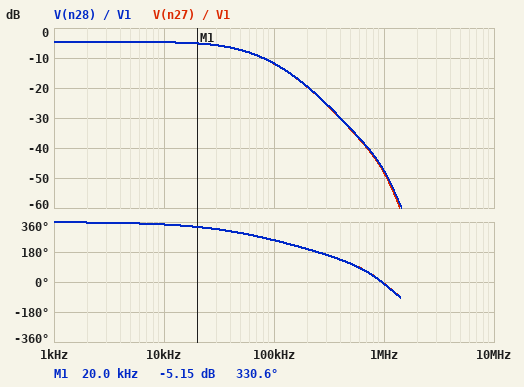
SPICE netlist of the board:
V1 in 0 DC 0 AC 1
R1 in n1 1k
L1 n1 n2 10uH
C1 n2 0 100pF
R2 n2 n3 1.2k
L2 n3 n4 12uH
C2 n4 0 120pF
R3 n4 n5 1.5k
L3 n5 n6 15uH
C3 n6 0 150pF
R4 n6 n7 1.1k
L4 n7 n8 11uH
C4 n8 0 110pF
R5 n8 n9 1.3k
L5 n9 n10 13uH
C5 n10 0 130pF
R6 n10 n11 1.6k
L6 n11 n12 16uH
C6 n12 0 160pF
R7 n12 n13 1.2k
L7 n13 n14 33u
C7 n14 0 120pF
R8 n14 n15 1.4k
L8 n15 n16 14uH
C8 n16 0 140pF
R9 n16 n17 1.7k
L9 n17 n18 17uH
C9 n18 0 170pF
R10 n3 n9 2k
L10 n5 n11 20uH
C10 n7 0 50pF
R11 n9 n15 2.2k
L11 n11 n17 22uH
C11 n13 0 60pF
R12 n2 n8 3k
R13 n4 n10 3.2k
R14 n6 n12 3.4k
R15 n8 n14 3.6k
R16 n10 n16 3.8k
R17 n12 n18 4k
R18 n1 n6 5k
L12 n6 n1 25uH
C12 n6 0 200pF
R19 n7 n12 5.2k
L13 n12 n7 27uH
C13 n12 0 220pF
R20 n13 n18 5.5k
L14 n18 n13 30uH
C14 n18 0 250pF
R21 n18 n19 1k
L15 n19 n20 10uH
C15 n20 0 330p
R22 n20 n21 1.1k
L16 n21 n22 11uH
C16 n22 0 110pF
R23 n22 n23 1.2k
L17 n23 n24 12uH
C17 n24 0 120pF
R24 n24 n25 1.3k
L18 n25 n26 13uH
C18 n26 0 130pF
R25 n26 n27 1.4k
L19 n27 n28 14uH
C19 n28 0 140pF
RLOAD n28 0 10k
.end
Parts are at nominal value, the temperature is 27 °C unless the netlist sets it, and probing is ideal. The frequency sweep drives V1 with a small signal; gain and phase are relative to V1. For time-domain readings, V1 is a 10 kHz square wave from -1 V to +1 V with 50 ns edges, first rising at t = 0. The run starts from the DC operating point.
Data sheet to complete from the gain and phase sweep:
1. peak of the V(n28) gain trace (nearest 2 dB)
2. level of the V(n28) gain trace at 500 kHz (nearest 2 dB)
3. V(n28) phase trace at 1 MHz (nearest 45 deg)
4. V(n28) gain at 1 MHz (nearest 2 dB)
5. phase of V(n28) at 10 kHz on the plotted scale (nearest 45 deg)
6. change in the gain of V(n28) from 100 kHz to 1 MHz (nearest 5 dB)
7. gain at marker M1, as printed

-4 dB
-34 dB
0 deg
-48 dB
360 deg
-35 dB
-5.15 dB
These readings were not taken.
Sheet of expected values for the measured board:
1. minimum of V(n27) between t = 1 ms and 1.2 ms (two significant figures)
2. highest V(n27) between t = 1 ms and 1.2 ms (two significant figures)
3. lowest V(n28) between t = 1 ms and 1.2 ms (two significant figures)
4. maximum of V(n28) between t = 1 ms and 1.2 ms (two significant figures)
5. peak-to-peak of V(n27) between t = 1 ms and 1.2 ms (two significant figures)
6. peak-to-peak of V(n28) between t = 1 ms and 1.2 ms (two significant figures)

-590 mV
590 mV
-590 mV
590 mV
1.2 V
1.2 V
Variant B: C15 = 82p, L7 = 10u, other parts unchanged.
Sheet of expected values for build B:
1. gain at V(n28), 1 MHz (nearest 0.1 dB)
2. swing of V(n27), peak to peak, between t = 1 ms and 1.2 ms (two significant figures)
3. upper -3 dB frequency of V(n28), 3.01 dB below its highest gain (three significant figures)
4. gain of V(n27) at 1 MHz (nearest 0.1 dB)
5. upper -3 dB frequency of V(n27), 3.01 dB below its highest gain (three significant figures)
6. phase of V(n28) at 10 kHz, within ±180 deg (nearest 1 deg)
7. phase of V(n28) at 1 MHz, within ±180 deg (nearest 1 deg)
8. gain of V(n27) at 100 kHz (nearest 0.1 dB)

-42.6 dB
1.2 V
58.7 kHz
-43.3 dB
58.6 kHz
-13 deg
19 deg
-11.1 dB
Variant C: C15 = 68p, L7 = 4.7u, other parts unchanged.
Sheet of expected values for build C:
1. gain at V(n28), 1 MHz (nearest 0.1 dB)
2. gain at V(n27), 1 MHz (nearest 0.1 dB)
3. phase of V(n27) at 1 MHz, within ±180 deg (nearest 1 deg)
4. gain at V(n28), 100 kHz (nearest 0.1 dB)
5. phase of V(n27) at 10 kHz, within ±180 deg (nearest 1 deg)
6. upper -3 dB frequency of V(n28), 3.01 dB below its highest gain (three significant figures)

-42.3 dB
-43.0 dB
22 deg
-11.0 dB
-13 deg
59.0 kHz
